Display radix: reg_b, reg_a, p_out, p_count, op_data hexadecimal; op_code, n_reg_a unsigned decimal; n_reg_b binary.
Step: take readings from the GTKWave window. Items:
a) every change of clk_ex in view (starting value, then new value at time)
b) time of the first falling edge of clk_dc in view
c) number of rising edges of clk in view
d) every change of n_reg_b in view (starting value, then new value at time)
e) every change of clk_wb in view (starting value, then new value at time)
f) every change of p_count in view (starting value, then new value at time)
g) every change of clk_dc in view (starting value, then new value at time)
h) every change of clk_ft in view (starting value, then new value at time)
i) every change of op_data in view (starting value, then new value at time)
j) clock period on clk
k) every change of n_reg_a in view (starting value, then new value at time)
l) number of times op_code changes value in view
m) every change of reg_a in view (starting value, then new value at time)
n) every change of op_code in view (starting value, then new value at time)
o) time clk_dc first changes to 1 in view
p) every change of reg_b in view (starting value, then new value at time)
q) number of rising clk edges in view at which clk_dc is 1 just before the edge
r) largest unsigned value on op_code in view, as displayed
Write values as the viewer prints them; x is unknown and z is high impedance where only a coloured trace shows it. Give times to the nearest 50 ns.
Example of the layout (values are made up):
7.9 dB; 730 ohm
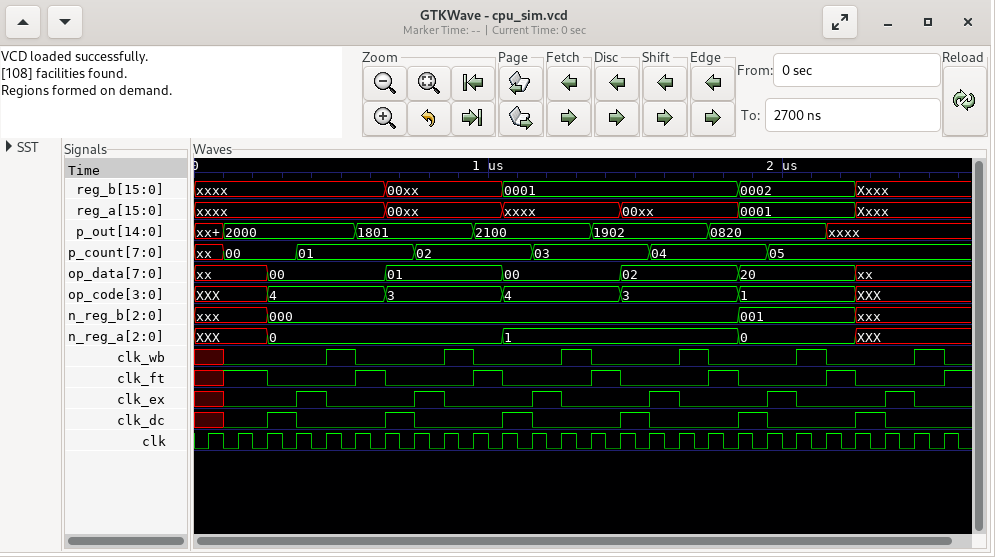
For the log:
x, 0 at 100 ns, 1 at 350 ns, 0 at 450 ns, 1 at 750 ns, 0 at 850 ns, 1 at 1150 ns, 0 at 1250 ns, 1 at 1550 ns, 0 at 1650 ns, 1 at 1950 ns, 0 at 2050 ns, 1 at 2350 ns, 0 at 2450 ns; 350 ns; 26; xxx, 000 at 250 ns, 001 at 1850 ns, xxx at 2250 ns; x, 0 at 100 ns, 1 at 450 ns, 0 at 550 ns, 1 at 850 ns, 0 at 950 ns, 1 at 1250 ns, 0 at 1350 ns, 1 at 1650 ns, 0 at 1750 ns, 1 at 2050 ns, 0 at 2150 ns, 1 at 2450 ns, 0 at 2550 ns; xx, 00 at 100 ns, 01 at 350 ns, 02 at 750 ns, 03 at 1150 ns, 04 at 1550 ns, 05 at 1950 ns; x, 0 at 100 ns, 1 at 250 ns, 0 at 350 ns, 1 at 650 ns, 0 at 750 ns, 1 at 1050 ns, 0 at 1150 ns, 1 at 1450 ns, 0 at 1550 ns, 1 at 1850 ns, 0 at 1950 ns, 1 at 2250 ns, 0 at 2350 ns; x, 1 at 100 ns, 0 at 250 ns, 1 at 550 ns, 0 at 650 ns, 1 at 950 ns, 0 at 1050 ns, 1 at 1350 ns, 0 at 1450 ns, 1 at 1750 ns, 0 at 1850 ns, 1 at 2150 ns, 0 at 2250 ns, 1 at 2550 ns; xx, 00 at 250 ns, 01 at 650 ns, 00 at 1050 ns, 02 at 1450 ns, 20 at 1850 ns, xx at 2250 ns; 100 ns; XXX, 0 at 250 ns, 1 at 1050 ns, 0 at 1850 ns, XXX at 2250 ns; 6; xxxx, 00xx at 650 ns, xxxx at 1050 ns, 00xx at 1450 ns, 0001 at 1850 ns, Xxxx at 2250 ns; XXX, 4 at 250 ns, 3 at 650 ns, 4 at 1050 ns, 3 at 1450 ns, 1 at 1850 ns, XXX at 2250 ns; 250 ns; xxxx, 00xx at 650 ns, 0001 at 1050 ns, 0002 at 1850 ns, Xxxx at 2250 ns; 6; 4
